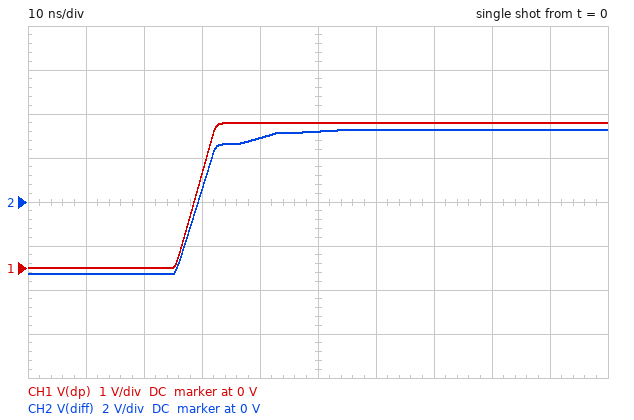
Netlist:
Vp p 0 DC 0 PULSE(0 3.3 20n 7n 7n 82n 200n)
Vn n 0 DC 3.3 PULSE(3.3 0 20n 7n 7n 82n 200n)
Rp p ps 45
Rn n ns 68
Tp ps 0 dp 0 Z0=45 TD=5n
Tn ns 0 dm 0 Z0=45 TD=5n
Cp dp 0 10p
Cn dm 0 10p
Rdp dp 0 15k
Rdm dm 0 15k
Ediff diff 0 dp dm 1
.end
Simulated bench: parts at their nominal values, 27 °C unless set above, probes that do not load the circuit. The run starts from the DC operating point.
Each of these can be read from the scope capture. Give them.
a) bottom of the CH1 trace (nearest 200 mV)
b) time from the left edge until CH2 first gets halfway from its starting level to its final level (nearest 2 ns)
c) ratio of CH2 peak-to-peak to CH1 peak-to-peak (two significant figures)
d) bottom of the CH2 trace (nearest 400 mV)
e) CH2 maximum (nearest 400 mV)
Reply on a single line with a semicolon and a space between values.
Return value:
0 V; 30 ns; 2.0; -3.2 V; 3.2 V
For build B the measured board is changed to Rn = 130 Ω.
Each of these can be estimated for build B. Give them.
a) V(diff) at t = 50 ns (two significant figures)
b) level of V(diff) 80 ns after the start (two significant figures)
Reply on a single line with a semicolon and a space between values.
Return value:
2.7 V; 3.2 V
